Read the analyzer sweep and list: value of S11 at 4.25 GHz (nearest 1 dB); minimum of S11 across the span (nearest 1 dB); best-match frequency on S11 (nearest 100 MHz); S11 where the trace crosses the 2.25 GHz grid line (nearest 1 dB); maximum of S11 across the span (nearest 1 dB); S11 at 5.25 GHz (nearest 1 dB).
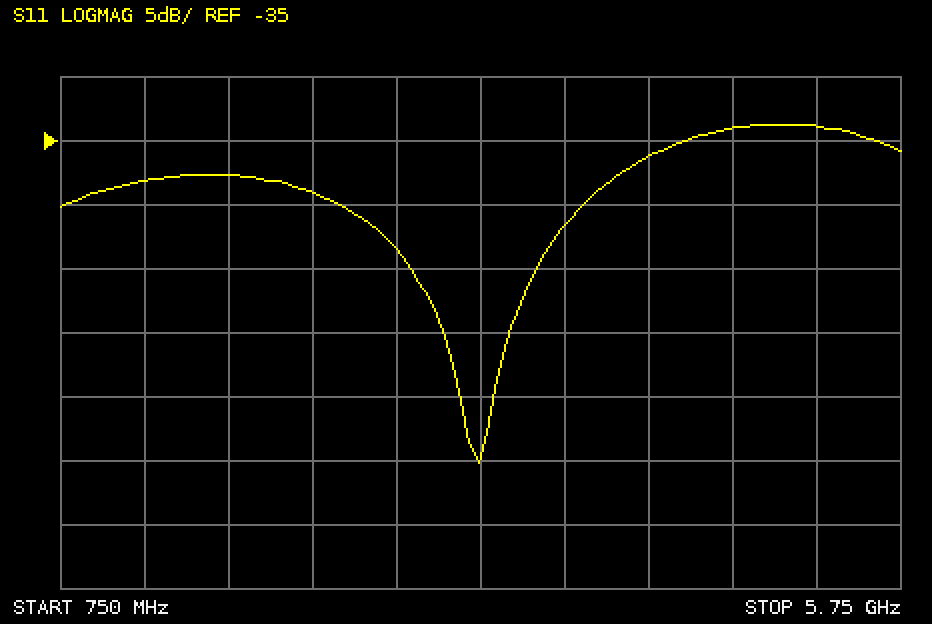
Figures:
-36 dB
-60 dB
3.2 GHz
-39 dB
-34 dB
-34 dB
